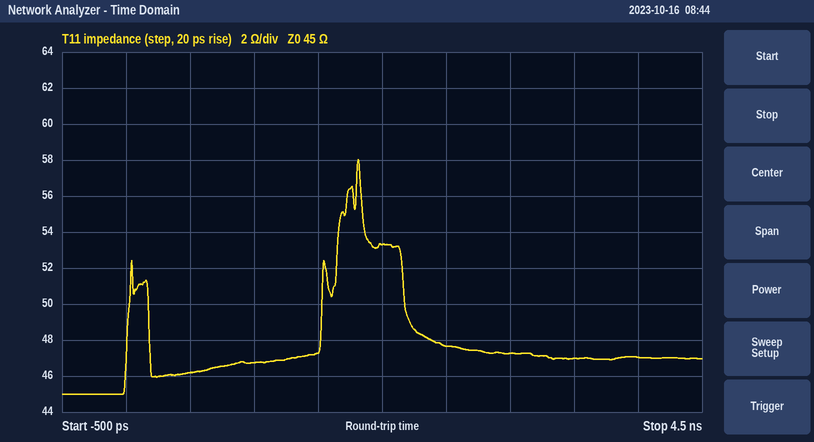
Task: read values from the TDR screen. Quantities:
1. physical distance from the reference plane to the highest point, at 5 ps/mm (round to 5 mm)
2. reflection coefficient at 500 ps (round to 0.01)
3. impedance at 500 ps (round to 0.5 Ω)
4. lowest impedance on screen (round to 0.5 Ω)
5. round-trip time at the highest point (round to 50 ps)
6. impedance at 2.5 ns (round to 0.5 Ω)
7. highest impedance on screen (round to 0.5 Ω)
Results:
180 mm
+0.01
46.0 Ω
45.0 Ω
1.80 ns
47.5 Ω
58.0 Ω
